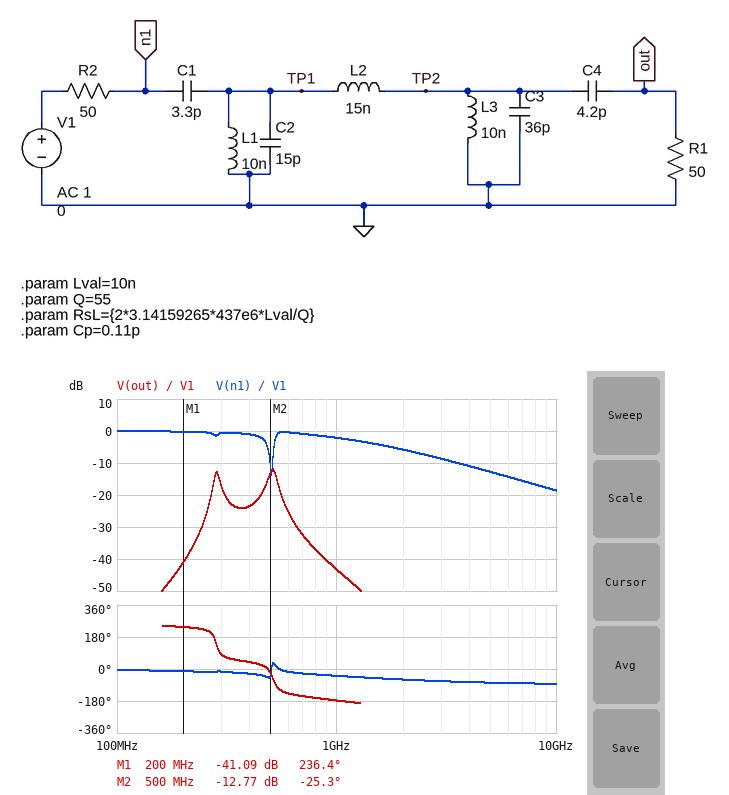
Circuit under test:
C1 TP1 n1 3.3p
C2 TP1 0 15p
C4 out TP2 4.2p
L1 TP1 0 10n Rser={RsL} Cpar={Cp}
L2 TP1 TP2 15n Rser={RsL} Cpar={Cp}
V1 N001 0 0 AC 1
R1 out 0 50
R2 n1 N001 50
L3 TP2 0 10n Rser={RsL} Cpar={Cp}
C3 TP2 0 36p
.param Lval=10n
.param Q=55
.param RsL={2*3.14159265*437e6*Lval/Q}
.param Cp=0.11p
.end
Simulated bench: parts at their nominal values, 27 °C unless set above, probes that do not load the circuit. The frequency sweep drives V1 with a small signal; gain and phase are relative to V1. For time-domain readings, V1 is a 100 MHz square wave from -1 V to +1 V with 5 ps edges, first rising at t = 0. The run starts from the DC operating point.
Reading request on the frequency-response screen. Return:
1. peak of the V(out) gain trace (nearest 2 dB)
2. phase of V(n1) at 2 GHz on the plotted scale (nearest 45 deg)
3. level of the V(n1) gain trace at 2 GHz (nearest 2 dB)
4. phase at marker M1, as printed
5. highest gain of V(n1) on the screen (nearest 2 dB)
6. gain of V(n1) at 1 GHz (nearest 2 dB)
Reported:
-12 dB
-45 deg
-6 dB
236.4 deg
0 dB
-2 dB
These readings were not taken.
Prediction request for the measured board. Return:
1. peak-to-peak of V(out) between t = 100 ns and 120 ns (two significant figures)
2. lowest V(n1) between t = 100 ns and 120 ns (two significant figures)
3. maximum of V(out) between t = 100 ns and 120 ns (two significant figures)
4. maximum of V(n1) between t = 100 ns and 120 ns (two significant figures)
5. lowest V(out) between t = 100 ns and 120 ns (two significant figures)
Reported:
230 mV
-1.2 V
120 mV
1.2 V
-120 mV
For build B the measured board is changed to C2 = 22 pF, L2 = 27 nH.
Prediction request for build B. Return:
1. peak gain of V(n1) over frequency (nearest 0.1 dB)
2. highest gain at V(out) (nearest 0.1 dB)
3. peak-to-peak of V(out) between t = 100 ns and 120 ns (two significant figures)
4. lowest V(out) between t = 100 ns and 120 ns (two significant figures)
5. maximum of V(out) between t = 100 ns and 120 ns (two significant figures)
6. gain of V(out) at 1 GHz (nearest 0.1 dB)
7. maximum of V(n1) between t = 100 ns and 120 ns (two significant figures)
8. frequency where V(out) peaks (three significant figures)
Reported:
0 dB
-11.2 dB
85 mV
-43 mV
43 mV
-53.3 dB
1.0 V
389 MHz
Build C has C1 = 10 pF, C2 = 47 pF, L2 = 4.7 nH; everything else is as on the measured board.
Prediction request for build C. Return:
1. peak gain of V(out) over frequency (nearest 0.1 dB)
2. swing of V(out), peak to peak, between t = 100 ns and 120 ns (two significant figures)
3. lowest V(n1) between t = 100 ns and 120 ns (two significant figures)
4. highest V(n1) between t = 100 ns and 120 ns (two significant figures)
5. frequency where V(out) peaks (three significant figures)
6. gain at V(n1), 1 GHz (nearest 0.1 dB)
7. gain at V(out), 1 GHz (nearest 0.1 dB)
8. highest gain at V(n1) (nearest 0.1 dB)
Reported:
-9.1 dB
150 mV
-1.1 V
1.1 V
550 MHz
-8.6 dB
-39.3 dB
0 dB
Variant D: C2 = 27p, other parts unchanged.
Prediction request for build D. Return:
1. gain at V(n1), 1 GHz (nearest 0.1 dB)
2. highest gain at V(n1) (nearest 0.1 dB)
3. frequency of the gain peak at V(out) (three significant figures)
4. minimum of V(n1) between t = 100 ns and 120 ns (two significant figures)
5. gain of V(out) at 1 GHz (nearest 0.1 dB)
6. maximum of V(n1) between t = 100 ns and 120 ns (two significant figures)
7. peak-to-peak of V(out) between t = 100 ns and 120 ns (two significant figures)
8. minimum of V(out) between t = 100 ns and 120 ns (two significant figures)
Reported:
-2.6 dB
0 dB
418 MHz
-1.0 V
-49.1 dB
1.0 V
93 mV
-46 mV
